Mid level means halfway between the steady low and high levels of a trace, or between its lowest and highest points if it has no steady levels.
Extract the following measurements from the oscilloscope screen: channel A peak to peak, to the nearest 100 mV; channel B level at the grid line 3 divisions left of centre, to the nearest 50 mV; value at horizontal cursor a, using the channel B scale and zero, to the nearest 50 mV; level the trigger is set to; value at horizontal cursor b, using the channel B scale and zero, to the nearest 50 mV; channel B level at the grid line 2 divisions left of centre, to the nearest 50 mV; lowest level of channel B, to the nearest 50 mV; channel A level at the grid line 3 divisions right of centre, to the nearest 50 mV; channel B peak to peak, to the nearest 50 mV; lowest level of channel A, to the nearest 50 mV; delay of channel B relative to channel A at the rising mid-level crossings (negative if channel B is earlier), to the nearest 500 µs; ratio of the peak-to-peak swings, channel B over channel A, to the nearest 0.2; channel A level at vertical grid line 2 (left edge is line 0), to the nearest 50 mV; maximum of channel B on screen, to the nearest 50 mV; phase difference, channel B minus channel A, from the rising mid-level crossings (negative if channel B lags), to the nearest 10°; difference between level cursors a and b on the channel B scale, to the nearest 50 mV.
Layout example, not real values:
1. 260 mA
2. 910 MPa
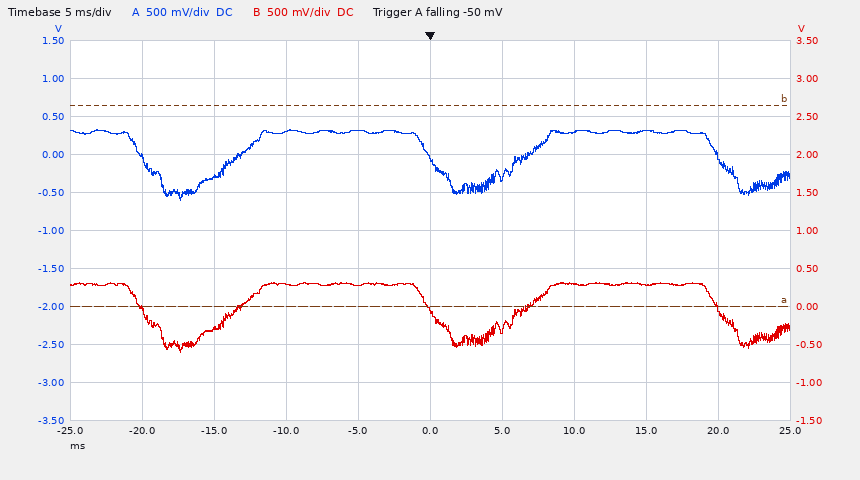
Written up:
1. 900 mV
2. -300 mV
3. 0 mV
4. -50 mV
5. 2.65 V
6. 300 mV
7. -600 mV
8. 300 mV
9. 900 mV
10. -600 mV
11. 0.0 ms
12. 1.0
13. -300 mV
14. 300 mV
15. 0°
16. 2.65 V
